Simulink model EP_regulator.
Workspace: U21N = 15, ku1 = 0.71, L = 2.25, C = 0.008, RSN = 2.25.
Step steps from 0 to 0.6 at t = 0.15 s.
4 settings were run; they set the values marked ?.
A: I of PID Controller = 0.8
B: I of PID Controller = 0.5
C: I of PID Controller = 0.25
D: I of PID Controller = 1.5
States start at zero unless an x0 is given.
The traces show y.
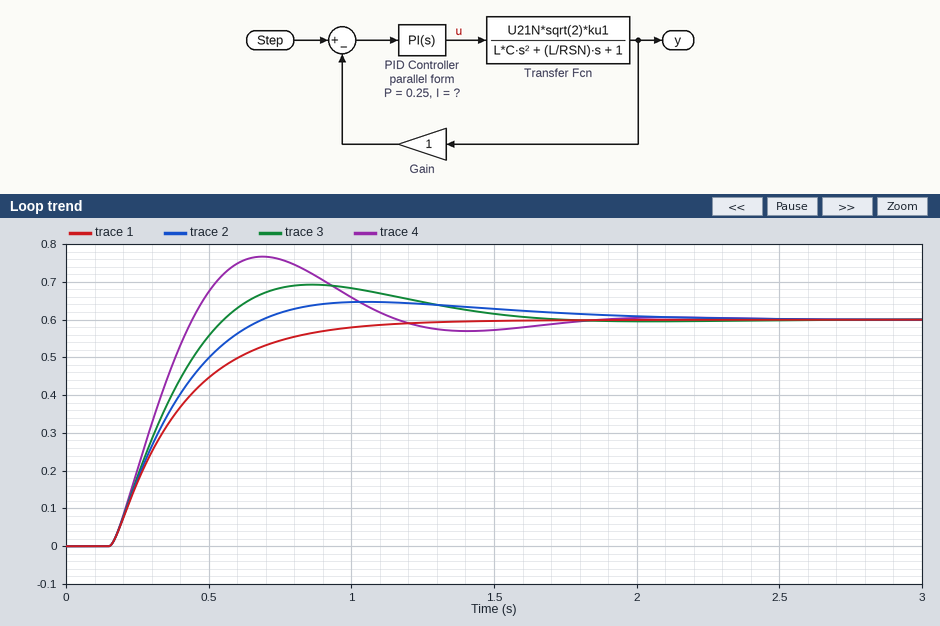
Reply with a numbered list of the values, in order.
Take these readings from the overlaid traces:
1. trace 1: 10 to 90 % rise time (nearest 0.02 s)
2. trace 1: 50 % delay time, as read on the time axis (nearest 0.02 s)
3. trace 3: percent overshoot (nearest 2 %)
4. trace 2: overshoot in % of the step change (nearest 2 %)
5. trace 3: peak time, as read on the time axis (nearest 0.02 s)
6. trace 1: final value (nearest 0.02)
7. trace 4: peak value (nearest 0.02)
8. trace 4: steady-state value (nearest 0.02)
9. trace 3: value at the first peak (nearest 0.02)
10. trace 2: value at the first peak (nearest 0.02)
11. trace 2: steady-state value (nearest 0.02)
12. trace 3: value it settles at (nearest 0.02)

1. 0.54 s
2. 0.34 s
3. 16 %
4. 8 %
5. 0.86 s
6. 0.60
7. 0.76
8. 0.60
9. 0.70
10. 0.64
11. 0.60
12. 0.60
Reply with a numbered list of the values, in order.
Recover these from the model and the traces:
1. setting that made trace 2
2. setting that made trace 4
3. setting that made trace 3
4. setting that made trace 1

1. B
2. D
3. A
4. C
